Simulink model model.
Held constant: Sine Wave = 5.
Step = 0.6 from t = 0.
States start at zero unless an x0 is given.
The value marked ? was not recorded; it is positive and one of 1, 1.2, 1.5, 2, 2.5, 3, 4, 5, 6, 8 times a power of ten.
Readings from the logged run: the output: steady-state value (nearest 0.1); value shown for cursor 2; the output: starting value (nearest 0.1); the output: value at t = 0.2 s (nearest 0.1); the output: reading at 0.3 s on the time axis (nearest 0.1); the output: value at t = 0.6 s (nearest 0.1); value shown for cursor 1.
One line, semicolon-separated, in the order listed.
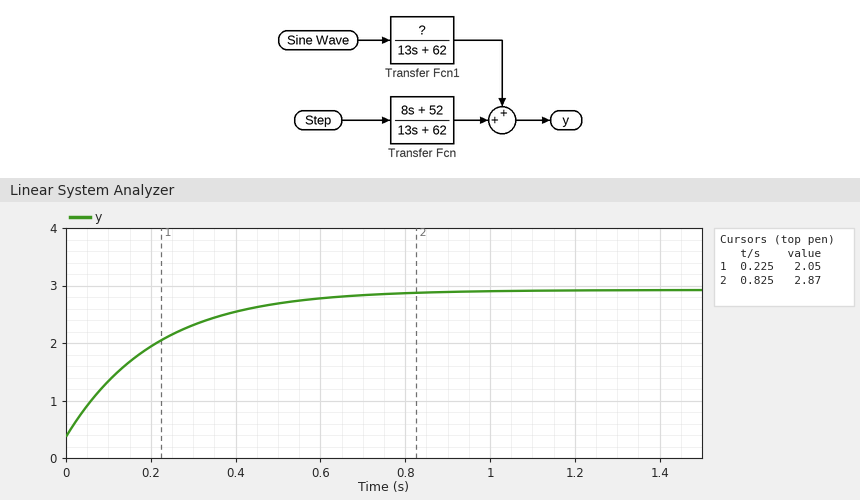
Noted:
2.9; 2.87; 0.4; 1.9; 2.3; 2.8; 2.05
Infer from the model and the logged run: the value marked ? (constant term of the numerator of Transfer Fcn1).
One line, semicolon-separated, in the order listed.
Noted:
30
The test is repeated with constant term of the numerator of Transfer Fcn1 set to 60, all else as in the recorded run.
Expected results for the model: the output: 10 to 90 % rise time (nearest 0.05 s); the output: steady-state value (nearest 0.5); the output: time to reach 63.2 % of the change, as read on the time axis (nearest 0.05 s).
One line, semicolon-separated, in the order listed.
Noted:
0.45 s; 5.5; 0.20 s
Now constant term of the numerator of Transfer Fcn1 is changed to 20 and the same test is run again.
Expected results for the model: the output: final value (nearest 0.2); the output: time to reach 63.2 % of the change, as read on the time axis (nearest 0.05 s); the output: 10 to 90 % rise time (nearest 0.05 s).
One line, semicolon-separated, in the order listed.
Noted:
2.2; 0.20 s; 0.45 s
